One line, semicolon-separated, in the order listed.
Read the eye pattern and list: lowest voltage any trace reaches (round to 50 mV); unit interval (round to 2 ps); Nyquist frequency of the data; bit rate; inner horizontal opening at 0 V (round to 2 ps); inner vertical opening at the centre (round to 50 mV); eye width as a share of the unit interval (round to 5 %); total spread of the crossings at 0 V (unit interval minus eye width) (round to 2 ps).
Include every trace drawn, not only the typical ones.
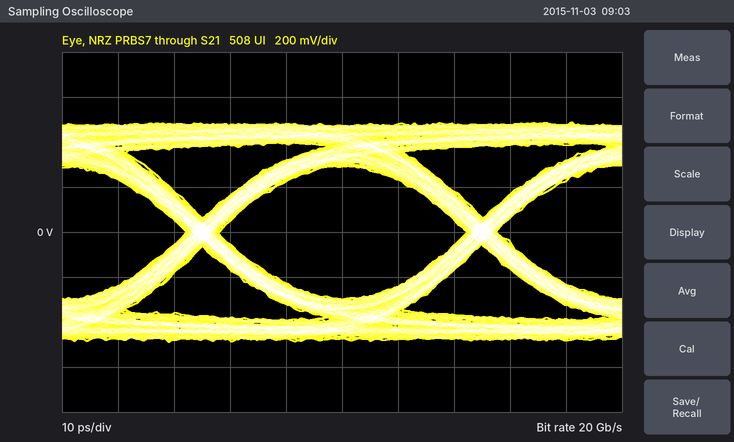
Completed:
-500 mV; 50 ps; 10 GHz; 20 Gb/s; 44 ps; 600 mV; 90 %; 6 ps
